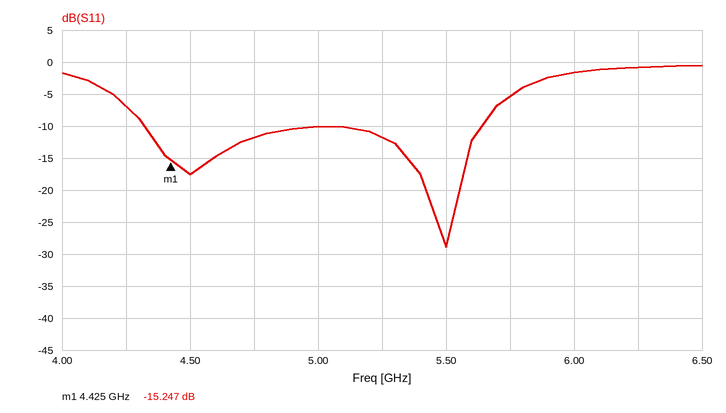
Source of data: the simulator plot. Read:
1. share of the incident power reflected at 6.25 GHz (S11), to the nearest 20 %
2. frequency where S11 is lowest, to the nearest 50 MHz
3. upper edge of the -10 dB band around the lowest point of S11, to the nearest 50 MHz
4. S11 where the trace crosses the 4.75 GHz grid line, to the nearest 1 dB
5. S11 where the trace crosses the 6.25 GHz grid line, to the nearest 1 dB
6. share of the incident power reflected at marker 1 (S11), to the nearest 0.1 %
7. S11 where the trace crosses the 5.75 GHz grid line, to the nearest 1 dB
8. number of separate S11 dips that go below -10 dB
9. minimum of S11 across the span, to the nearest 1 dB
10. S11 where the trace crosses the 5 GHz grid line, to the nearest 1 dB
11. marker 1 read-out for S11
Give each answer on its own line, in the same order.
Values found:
80 %
5.50 GHz
5.65 GHz
-12 dB
-1 dB
3.0 %
-5 dB
2
-29 dB
-10 dB
-15.247 dB
